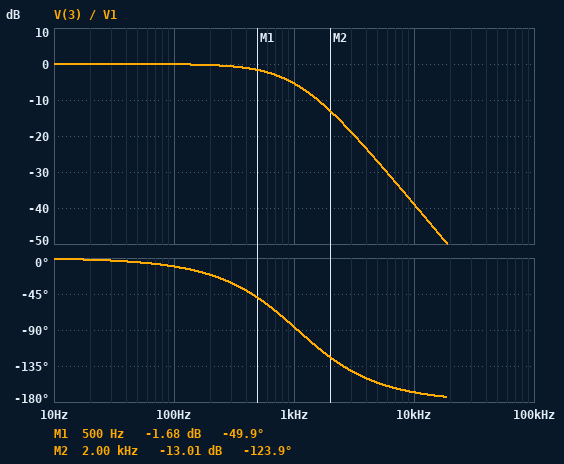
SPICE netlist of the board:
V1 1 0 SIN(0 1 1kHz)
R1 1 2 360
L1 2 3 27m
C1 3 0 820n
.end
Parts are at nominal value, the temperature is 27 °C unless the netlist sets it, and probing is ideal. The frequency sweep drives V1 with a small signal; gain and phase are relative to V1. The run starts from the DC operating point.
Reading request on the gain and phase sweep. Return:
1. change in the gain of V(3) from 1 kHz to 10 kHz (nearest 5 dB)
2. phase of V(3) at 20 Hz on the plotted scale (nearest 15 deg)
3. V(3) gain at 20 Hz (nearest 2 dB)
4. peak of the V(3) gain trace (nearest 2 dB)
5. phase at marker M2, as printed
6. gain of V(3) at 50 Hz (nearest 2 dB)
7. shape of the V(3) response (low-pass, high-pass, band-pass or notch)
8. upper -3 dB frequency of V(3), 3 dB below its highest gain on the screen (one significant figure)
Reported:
-35 dB
0 deg
0 dB
0 dB
-123.9 deg
0 dB
low-pass
700 Hz
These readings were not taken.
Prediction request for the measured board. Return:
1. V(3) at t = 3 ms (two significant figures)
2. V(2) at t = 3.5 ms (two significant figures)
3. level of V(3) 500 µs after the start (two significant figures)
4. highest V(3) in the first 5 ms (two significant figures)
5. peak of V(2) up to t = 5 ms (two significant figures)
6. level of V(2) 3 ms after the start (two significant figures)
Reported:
-540 mV
68 mV
610 mV
620 mV
360 mV
-68 mV
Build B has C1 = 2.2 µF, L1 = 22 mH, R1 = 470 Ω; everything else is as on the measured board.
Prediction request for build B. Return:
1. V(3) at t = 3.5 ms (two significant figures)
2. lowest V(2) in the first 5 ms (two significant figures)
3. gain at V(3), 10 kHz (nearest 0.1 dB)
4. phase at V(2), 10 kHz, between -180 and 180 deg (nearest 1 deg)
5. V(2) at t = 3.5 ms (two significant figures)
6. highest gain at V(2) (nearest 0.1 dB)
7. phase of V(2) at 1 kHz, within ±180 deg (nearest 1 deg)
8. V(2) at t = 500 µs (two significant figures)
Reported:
160 mV
-140 mV
-46.1 dB
19 deg
-130 mV
0 dB
82 deg
-33 mV
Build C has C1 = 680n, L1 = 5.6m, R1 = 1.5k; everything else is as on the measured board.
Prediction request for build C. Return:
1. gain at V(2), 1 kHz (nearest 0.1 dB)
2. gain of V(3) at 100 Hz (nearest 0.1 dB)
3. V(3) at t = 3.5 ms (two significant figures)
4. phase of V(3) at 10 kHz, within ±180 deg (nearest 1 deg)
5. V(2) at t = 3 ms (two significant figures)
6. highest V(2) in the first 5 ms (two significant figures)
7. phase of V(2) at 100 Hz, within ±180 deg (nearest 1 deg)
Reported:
-17.6 dB
-1.5 dB
160 mV
-102 deg
-120 mV
230 mV
-33 deg
